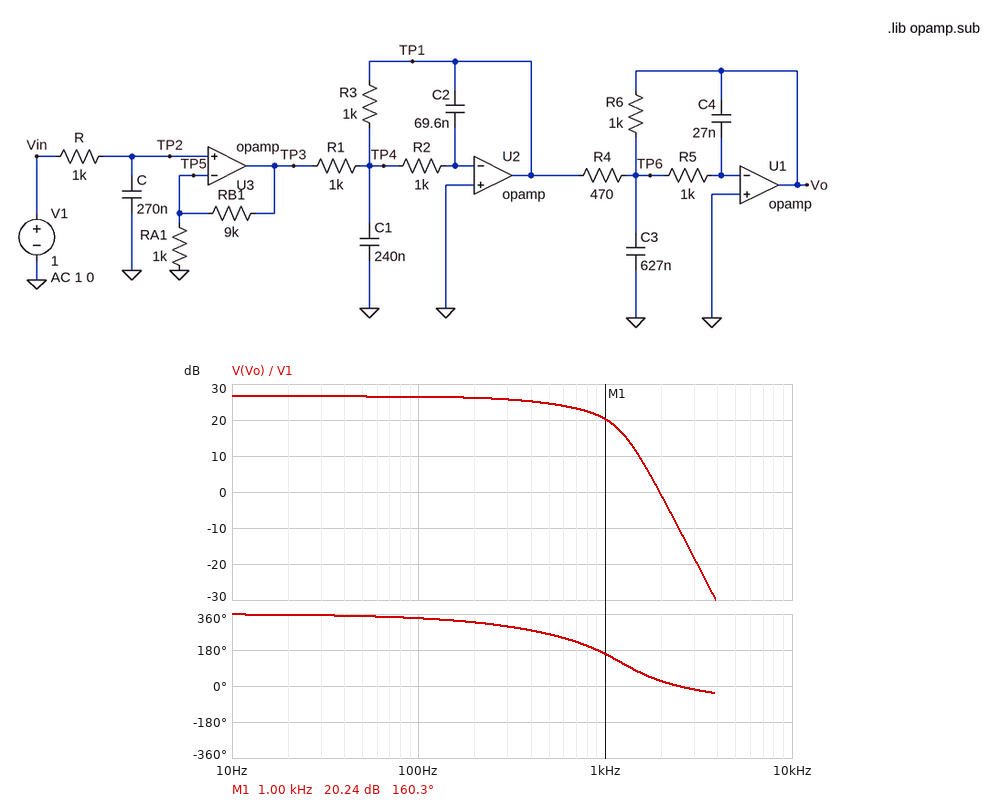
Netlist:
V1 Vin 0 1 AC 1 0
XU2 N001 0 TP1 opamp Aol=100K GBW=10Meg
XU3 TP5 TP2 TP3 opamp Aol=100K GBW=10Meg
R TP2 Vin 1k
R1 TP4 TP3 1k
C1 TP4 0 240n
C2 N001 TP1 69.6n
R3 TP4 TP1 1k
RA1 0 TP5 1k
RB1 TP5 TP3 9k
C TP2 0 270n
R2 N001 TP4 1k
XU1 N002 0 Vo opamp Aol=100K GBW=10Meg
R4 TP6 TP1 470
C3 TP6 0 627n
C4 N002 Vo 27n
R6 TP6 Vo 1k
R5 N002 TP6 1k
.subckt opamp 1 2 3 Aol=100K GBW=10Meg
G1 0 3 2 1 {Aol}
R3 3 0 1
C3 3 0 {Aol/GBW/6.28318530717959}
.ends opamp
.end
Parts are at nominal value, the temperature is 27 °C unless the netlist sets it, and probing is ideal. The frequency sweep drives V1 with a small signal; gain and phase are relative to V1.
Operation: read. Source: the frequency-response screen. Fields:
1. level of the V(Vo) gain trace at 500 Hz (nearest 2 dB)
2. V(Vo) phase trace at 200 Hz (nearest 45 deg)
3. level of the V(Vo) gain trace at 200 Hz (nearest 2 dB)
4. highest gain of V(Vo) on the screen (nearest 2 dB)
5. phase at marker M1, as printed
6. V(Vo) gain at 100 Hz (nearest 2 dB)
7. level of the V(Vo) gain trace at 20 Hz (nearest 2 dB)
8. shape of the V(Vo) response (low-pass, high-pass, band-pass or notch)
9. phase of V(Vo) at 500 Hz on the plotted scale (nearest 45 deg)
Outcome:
24 dB
315 deg
26 dB
26 dB
160.3 deg
26 dB
26 dB
low-pass
270 deg
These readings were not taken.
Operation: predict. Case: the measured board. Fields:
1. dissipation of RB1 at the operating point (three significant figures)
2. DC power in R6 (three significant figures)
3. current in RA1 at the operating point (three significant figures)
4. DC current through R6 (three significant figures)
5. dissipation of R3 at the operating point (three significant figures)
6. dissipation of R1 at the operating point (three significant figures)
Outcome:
9.00 mW
453 mW
1.00 mA
21.3 mA
100 mW
100 mW
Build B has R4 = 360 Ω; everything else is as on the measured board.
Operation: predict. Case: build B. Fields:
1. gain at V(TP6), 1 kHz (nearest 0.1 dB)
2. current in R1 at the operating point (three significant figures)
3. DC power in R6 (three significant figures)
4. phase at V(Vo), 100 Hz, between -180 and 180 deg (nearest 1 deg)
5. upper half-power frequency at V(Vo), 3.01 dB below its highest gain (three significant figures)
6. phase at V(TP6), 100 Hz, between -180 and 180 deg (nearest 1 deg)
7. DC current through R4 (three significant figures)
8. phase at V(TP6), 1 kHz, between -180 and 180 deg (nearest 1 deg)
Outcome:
6.1 dB
10.0 mA
771 mW
-22 deg
603 Hz
-112 deg
27.8 mA
67 deg
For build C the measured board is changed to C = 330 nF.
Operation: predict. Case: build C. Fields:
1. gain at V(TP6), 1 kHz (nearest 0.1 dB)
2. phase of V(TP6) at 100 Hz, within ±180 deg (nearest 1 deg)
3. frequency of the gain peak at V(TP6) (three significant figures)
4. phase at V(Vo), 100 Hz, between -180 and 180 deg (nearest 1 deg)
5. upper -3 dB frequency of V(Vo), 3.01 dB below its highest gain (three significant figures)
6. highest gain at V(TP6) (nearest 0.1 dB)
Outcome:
3.5 dB
-113 deg
845 Hz
-23 deg
525 Hz
3.9 dB
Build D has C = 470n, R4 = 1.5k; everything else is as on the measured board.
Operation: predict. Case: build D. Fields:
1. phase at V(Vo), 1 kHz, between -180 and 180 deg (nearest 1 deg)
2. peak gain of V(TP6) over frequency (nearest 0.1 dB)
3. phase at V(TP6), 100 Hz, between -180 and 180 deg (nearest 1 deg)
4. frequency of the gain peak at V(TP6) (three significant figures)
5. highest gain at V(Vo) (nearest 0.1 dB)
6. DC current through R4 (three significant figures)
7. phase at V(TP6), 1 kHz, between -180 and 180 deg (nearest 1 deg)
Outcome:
159 deg
-6.4 dB
-117 deg
1.03 kHz
16.5 dB
6.67 mA
69 deg
